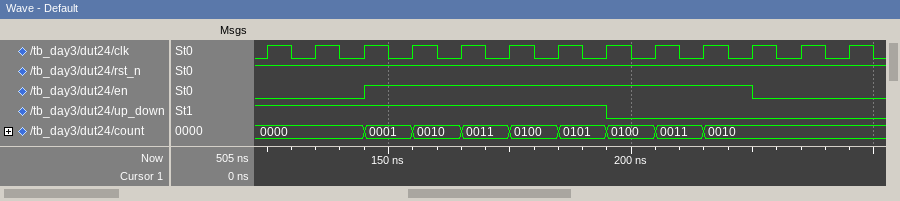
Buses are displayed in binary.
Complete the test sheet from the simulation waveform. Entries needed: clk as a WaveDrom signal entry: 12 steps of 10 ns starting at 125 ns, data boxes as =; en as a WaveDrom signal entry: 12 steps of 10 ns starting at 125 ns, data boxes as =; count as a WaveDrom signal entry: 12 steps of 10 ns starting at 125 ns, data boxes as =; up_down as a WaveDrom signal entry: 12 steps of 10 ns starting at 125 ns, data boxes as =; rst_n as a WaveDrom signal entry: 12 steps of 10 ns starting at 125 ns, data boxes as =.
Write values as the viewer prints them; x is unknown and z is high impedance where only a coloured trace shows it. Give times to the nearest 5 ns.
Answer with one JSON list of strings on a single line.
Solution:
["{name: 'clk', wave: 'p...........'}", "{name: 'en', wave: '0.1.......0.'}", "{name: 'count', wave: '=.========..', data: '0000 0001 0010 0011 0100 0101 0100 0011 0010'}", "{name: 'up_down', wave: '1......0....'}", "{name: 'rst_n', wave: '1...........'}"]
